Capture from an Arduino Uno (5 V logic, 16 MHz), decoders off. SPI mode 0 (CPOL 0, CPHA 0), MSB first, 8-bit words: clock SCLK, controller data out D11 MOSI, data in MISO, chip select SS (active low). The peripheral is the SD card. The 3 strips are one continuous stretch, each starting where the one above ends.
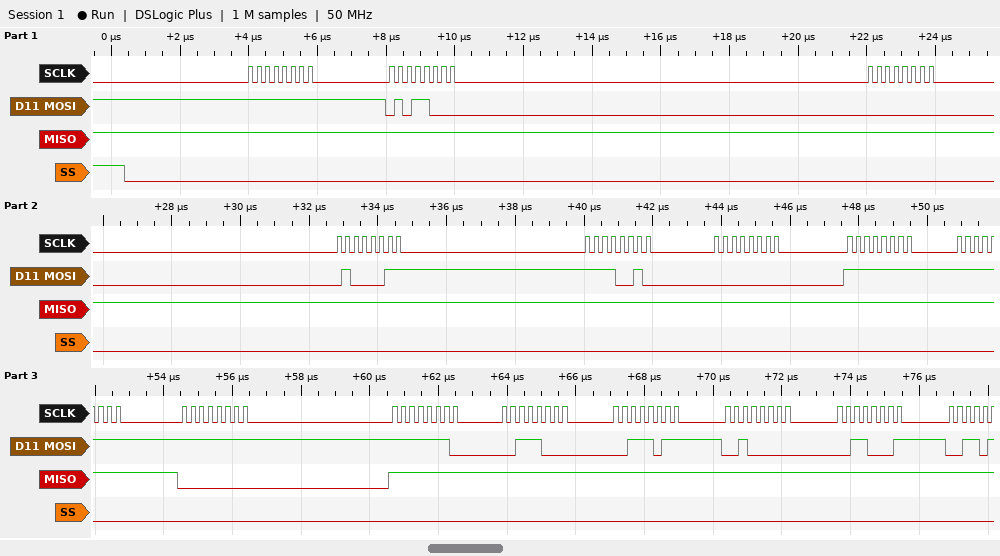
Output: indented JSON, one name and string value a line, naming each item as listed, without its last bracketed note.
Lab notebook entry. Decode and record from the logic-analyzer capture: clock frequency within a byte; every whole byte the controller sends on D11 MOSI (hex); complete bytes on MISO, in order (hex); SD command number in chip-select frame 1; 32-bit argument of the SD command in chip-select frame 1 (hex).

{
  "clock frequency within a byte": "4 MHz",
  "every whole byte the controller sends on D11 MOSI": "FF 58 00 43 F2 00 FF FF FF FE 38 3B 20 31",
  "complete bytes on MISO, in order": "FF FF FF FF FF FF FF FF 00 FF FF FF FF FF",
  "SD command number in chip-select frame 1": "CMD24",
  "32-bit argument of the SD command in chip-select frame 1": "0x0043F200"
}
